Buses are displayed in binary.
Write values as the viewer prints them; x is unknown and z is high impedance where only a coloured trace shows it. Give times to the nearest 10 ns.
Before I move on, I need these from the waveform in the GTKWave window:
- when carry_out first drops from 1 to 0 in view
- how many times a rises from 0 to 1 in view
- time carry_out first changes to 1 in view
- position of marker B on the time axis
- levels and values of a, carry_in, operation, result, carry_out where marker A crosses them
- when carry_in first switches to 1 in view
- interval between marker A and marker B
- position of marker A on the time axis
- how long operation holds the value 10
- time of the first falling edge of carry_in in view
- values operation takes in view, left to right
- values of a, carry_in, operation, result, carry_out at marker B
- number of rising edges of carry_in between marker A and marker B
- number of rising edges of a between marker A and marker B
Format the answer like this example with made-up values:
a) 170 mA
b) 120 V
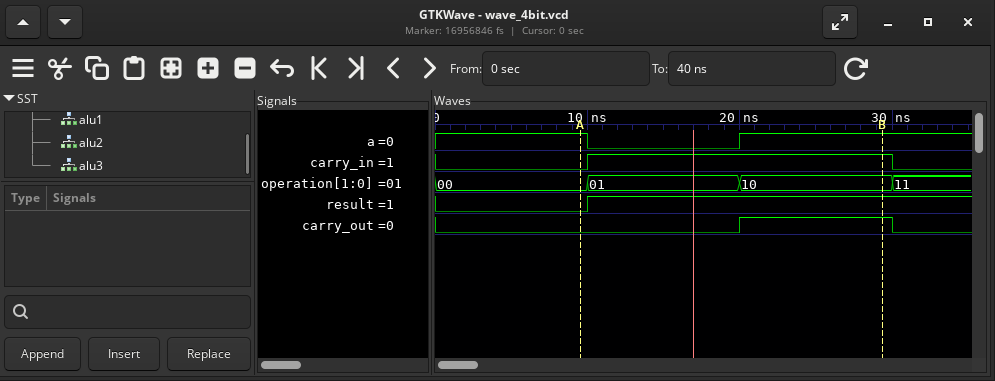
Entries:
a) 30 ns
b) 1
c) 20 ns
d) 30 ns
e) a=1, carry_in=0, operation=00, result=0, carry_out=0
f) 10 ns
g) 20 ns
h) 10 ns
i) 10 ns
j) 30 ns
k) 00, 01, 10, 11
l) a=1, carry_in=1, operation=10, result=1, carry_out=1
m) 1
n) 1
